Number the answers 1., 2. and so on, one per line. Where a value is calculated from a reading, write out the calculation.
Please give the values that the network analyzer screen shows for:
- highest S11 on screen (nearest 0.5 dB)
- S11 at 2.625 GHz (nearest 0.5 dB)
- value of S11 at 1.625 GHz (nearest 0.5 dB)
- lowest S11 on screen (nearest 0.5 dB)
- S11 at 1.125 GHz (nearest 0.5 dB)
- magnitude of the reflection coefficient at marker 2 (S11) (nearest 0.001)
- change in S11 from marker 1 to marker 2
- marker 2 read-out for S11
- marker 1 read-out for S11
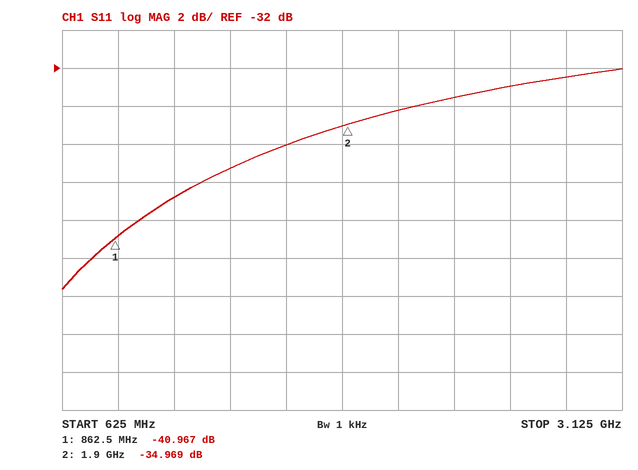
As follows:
1. -32.0 dB
2. -33.0 dB
3. -36.0 dB
4. -43.5 dB
5. -39.0 dB
6. 10^(-34.969/20) ≈ 0.018
7. -34.969 − (-40.967) = 5.998 dB
8. -34.969 dB
9. -40.967 dB
